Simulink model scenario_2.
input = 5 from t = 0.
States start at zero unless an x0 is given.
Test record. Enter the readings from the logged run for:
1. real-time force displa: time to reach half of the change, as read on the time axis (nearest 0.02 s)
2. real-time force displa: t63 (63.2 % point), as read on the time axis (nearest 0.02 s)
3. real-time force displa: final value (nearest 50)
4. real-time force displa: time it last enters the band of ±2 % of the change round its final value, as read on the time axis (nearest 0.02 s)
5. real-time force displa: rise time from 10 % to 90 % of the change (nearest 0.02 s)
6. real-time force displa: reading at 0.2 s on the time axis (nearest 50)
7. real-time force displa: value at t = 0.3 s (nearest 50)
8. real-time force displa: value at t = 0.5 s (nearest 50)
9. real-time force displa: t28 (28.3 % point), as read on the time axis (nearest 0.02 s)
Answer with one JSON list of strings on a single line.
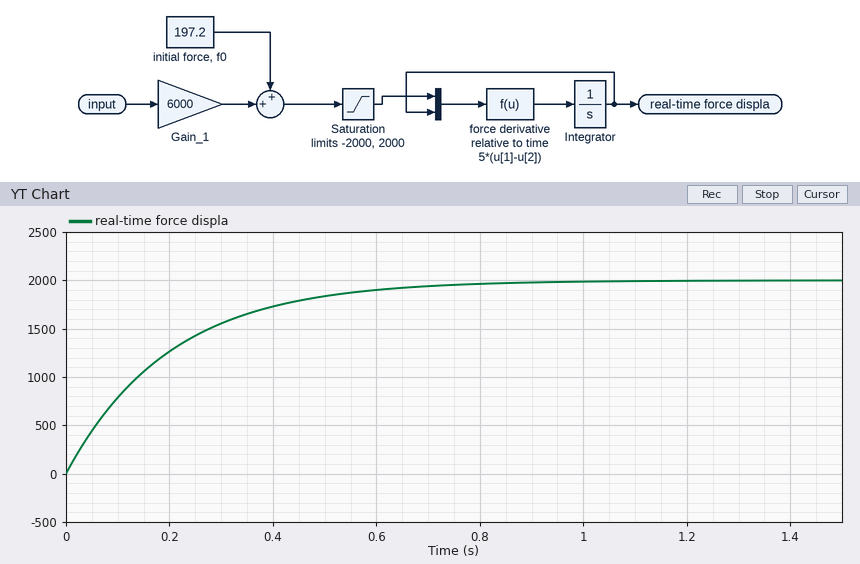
["0.14 s", "0.20 s", "2000", "0.78 s", "0.44 s", "1250", "1550", "1850", "0.06 s"]
